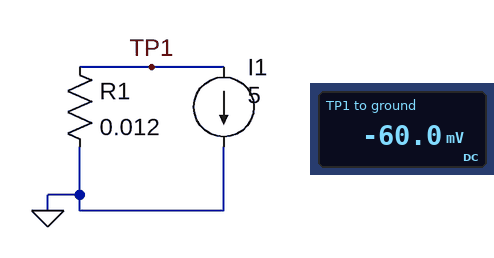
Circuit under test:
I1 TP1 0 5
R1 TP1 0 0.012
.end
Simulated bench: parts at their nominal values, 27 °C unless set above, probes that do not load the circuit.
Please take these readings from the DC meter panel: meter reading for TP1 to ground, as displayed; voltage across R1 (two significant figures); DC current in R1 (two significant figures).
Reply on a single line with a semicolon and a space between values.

-60.0 mV; 60 mV; 5.0 A
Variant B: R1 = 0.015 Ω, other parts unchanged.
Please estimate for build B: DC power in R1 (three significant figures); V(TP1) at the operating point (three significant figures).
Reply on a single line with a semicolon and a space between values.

375 mW; -75.0 mV
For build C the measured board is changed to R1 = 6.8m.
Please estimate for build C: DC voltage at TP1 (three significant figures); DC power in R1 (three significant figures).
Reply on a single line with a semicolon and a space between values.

-34.0 mV; 170 mW
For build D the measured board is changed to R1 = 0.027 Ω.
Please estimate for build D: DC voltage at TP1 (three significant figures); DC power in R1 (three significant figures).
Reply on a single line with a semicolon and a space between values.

-135 mV; 675 mW
